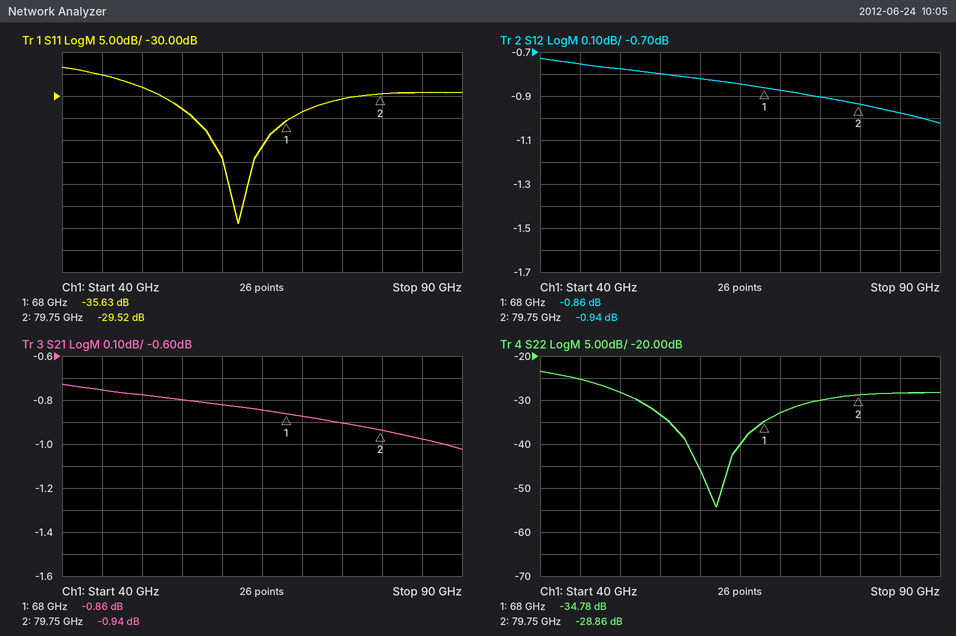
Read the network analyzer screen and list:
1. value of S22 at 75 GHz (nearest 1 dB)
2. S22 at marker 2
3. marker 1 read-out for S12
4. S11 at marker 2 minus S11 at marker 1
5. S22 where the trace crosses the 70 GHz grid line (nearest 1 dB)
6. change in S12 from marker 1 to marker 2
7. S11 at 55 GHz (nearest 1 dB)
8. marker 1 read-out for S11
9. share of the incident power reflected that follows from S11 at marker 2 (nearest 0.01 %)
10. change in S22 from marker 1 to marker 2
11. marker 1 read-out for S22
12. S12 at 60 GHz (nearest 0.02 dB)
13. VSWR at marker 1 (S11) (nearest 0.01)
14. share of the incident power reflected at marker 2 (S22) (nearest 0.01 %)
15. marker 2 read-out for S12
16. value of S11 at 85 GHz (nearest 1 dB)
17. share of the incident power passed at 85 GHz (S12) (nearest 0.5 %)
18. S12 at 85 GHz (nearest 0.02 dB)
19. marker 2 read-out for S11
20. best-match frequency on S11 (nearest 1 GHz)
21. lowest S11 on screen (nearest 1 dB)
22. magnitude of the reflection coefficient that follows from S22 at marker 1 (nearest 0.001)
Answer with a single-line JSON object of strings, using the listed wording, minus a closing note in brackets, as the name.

{"value of S22 at 75 GHz": "-30 dB", "S22 at marker 2": "-28.86 dB", "marker 1 read-out for S12": "-0.86 dB", "S11 at marker 2 minus S11 at marker 1": "6.11 dB", "S22 where the trace crosses the 70 GHz grid line": "-33 dB", "change in S12 from marker 1 to marker 2": "-0.08 dB", "S11 at 55 GHz": "-33 dB", "marker 1 read-out for S11": "-35.63 dB", "share of the incident power reflected that follows from S11 at marker 2": "0.11 %", "change in S22 from marker 1 to marker 2": "5.92 dB", "marker 1 read-out for S22": "-34.78 dB", "S12 at 60 GHz": "-0.82 dB", "VSWR at marker 1 (S11)": "1.03", "share of the incident power reflected at marker 2 (S22)": "0.13 %", "marker 2 read-out for S12": "-0.94 dB", "value of S11 at 85 GHz": "-29 dB", "share of the incident power passed at 85 GHz (S12)": "80.0 %", "S12 at 85 GHz": "-0.98 dB", "marker 2 read-out for S11": "-29.52 dB", "best-match frequency on S11": "62 GHz", "lowest S11 on screen": "-59 dB", "magnitude of the reflection coefficient that follows from S22 at marker 1": "0.018"}
